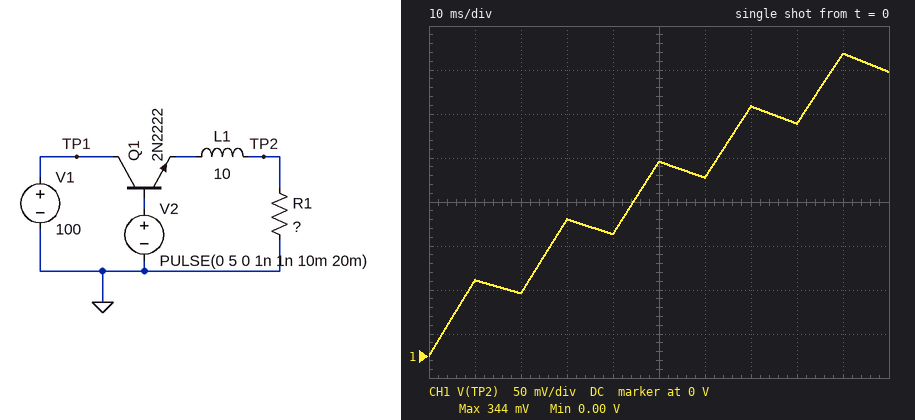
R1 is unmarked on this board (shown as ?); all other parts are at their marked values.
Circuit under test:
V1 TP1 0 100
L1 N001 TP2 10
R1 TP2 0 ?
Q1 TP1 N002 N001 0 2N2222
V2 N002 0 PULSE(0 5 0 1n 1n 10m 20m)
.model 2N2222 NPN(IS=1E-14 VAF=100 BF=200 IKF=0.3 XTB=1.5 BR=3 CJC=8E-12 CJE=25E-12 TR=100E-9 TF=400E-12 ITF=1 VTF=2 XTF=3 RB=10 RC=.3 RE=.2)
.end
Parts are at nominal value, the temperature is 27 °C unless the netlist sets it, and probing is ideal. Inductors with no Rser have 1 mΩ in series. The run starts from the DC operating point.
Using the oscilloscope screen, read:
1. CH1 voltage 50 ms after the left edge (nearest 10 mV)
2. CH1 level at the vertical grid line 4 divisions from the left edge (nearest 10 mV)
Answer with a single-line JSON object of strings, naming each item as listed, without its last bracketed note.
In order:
{"CH1 voltage 50 ms after the left edge": "220 mV", "CH1 level at the vertical grid line 4 divisions from the left edge": "140 mV"}
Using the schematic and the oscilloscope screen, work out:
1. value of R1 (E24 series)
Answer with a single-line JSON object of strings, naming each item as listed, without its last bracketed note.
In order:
{"value of R1": "20 Ω"}
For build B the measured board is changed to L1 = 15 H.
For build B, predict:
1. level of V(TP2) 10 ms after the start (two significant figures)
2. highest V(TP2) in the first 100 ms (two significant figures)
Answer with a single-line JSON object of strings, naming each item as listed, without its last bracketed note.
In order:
{"level of V(TP2) 10 ms after the start": "58 mV", "highest V(TP2) in the first 100 ms": "240 mV"}
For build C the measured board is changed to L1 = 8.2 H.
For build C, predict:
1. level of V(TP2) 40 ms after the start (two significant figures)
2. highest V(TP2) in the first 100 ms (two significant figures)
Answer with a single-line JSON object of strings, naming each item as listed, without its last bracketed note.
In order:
{"level of V(TP2) 40 ms after the start": "170 mV", "highest V(TP2) in the first 100 ms": "410 mV"}
